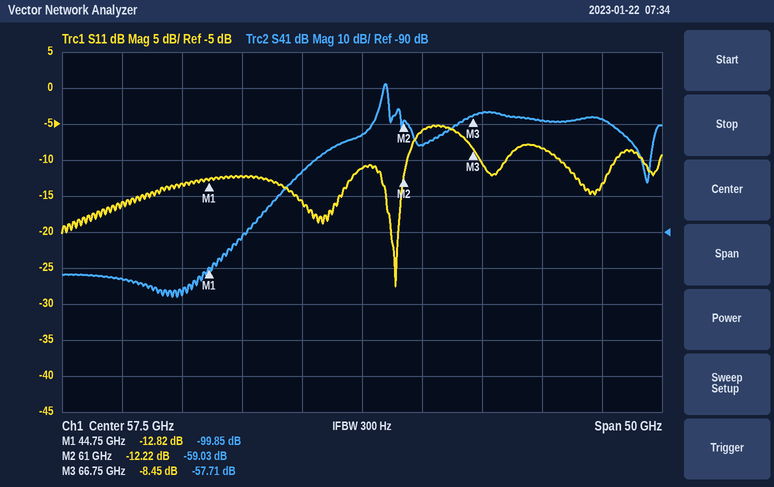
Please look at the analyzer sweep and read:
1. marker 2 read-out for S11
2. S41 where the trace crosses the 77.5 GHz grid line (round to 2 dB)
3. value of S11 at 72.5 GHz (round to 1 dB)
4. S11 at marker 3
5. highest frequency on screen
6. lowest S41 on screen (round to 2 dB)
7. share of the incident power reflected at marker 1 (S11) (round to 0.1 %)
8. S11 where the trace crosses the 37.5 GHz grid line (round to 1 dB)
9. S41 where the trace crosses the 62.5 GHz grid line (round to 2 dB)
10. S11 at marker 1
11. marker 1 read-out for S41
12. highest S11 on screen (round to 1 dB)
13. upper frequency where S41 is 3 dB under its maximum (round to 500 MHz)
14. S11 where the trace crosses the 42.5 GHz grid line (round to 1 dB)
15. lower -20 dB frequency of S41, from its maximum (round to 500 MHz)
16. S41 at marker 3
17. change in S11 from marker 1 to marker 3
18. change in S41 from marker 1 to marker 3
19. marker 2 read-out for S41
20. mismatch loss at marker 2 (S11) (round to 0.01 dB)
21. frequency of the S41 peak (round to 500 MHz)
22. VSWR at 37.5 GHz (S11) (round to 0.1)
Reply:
-12.22 dB
-58 dB
-8 dB
-8.45 dB
82.5 GHz
-108 dB
5.2 %
-16 dB
-66 dB
-12.82 dB
-99.85 dB
-5 dB
59.5 GHz
-13 dB
54.0 GHz
-57.71 dB
4.37 dB
42.14 dB
-59.03 dB
0.27 dB
59.5 GHz
1.4
